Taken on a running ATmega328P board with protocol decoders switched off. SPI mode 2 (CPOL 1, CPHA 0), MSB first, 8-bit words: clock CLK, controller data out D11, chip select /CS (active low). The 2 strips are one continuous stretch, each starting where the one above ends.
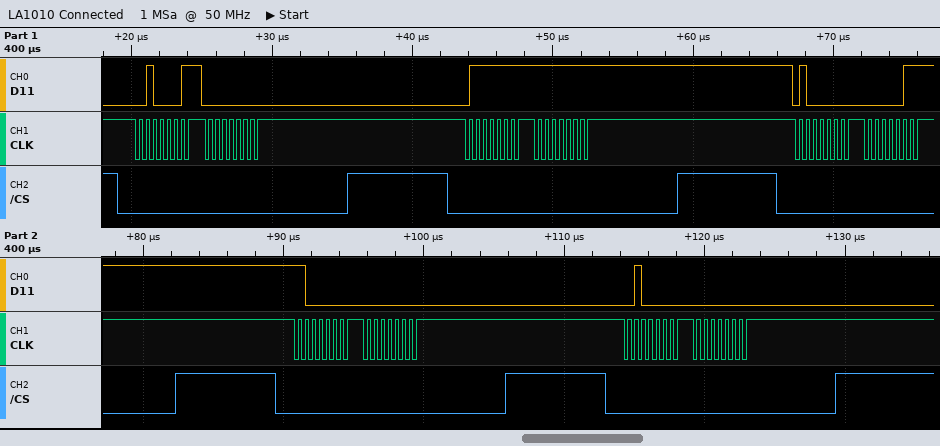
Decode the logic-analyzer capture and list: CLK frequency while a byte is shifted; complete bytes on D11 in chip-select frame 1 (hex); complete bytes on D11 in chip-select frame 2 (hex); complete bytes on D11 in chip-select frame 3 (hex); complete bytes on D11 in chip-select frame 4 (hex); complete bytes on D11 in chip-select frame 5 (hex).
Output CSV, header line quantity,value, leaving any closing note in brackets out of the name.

quantity,value
CLK frequency while a byte is shifted,2 MHz
complete bytes on D11 in chip-select frame 1,21 00
complete bytes on D11 in chip-select frame 2,7F FF
complete bytes on D11 in chip-select frame 3,40 03
complete bytes on D11 in chip-select frame 4,C0 00
complete bytes on D11 in chip-select frame 5,20 00
